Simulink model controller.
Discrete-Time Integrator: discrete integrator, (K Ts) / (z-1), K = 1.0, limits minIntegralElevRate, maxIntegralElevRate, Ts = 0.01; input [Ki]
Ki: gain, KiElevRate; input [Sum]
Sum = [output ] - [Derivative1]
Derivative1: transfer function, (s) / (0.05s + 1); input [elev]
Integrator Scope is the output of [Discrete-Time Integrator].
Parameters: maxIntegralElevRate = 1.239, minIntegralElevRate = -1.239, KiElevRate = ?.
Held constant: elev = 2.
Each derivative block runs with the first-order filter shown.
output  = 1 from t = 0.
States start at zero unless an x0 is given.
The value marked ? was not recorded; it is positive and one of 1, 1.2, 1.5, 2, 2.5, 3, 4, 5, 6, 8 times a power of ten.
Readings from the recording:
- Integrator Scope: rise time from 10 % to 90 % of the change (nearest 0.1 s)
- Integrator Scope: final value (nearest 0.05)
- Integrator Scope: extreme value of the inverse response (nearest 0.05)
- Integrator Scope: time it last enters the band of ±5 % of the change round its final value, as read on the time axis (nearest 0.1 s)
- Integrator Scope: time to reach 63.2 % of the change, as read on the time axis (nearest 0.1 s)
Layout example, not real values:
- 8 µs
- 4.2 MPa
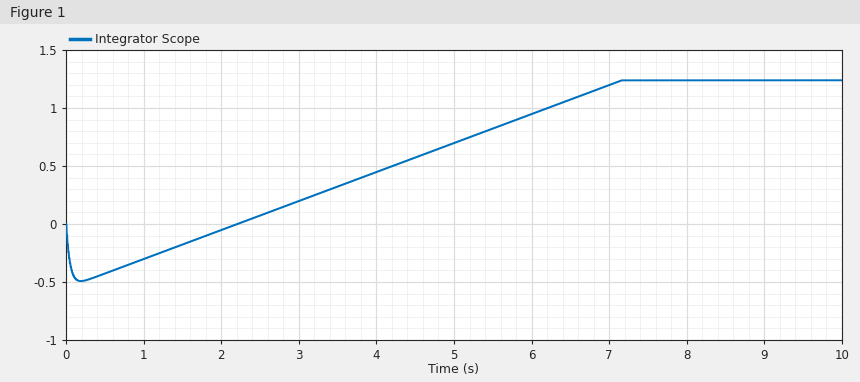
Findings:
- 4.0 s
- 1.25
- -0.50
- 6.9 s
- 5.3 s
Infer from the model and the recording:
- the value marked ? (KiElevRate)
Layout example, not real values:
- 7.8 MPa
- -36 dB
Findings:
- 0.25
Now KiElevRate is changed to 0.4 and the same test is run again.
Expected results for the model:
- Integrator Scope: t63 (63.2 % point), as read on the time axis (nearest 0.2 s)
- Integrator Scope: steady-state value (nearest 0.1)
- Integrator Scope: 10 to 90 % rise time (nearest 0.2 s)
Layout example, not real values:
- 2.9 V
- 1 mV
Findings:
- 4.2 s
- 1.2
- 2.4 s
